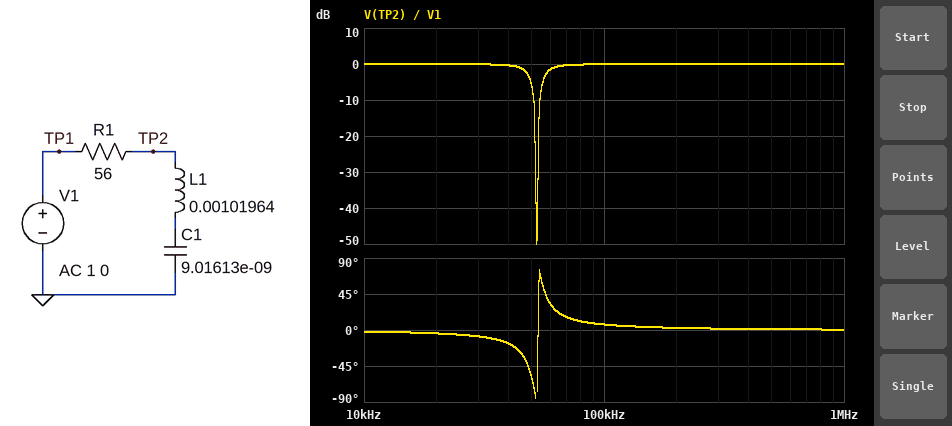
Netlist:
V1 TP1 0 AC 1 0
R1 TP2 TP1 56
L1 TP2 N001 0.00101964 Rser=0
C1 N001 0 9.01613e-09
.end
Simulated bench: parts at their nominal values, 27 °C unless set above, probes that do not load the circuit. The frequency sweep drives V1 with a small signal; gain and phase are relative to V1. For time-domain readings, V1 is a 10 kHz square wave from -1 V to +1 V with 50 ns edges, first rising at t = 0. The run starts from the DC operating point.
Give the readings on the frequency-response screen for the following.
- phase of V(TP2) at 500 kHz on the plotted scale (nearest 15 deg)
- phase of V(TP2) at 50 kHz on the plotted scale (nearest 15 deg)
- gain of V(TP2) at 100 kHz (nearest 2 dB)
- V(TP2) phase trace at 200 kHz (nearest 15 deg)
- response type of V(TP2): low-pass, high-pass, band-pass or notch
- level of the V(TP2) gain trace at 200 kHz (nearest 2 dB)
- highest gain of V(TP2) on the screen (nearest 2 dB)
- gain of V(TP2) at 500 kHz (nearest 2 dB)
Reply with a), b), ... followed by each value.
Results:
a) 0 deg
b) -60 deg
c) 0 dB
d) 0 deg
e) notch
f) 0 dB
g) 0 dB
h) 0 dB
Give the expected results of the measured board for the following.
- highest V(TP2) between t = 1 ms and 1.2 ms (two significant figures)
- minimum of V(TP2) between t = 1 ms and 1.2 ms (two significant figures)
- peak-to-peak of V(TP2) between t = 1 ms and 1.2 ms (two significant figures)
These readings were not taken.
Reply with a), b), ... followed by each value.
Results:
a) 1.3 V
b) -1.3 V
c) 2.6 V
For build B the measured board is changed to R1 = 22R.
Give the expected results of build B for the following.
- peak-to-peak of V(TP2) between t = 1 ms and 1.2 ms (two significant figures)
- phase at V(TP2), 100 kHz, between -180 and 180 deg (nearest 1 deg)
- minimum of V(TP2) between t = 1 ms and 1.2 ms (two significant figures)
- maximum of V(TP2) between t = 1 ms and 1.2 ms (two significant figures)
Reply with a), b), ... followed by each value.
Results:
a) 2.3 V
b) 3 deg
c) -1.2 V
d) 1.2 V
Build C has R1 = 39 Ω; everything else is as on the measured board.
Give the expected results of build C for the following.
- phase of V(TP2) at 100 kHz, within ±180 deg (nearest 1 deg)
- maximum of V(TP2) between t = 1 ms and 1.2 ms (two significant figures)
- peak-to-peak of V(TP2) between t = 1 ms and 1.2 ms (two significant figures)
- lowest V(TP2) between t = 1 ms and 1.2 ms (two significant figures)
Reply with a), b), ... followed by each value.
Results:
a) 5 deg
b) 1.2 V
c) 2.5 V
d) -1.2 V
